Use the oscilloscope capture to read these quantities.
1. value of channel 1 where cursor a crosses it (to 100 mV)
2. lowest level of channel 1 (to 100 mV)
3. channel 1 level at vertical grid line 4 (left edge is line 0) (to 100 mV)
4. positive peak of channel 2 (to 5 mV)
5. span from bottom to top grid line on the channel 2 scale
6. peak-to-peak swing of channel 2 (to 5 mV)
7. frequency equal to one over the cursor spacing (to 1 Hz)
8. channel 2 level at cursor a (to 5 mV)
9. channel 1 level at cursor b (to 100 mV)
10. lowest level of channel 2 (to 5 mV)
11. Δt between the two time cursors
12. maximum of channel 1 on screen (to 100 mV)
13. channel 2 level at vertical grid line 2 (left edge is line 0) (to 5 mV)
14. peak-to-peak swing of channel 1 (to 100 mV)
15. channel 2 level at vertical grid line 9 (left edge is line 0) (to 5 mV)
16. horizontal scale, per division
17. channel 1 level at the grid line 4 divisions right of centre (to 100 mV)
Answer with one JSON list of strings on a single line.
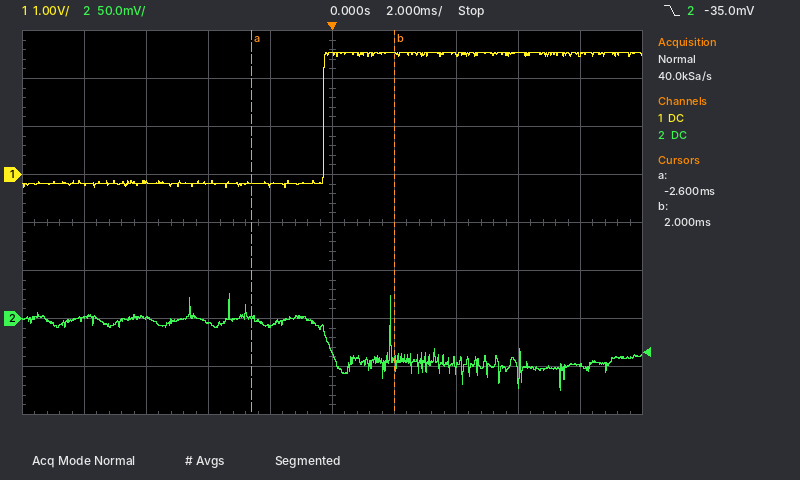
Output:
["-200 mV", "-300 mV", "-200 mV", "25 mV", "400 mV", "100 mV", "217 Hz", "0 mV", "2.5 V", "-75 mV", "4.6 ms", "2.5 V", "0 mV", "2.8 V", "-50 mV", "2 ms", "2.5 V"]
